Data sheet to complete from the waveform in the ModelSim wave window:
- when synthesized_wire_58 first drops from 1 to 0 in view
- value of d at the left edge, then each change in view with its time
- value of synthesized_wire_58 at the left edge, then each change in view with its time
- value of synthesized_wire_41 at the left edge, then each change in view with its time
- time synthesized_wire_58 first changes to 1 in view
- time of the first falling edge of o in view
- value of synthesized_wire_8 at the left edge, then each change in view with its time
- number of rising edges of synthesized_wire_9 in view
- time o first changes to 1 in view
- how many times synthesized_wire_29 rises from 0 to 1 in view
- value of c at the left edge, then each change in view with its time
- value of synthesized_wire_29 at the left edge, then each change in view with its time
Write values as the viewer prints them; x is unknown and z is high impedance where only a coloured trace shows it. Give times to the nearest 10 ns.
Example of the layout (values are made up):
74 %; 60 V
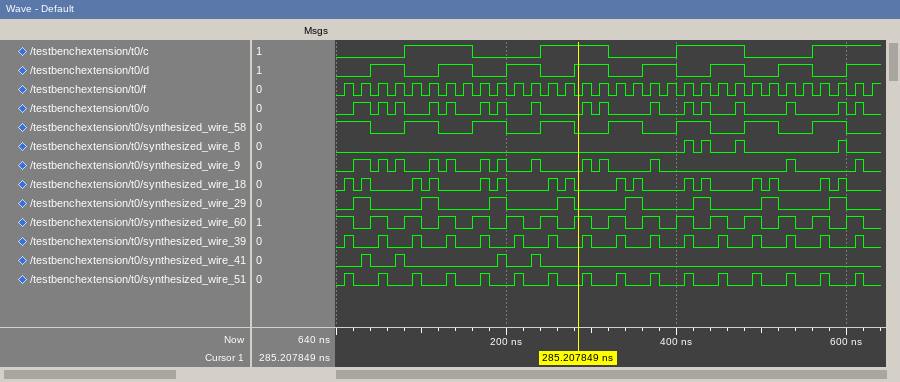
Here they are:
40 ns; 0, 1 at 40 ns, 0 at 80 ns, 1 at 120 ns, 0 at 160 ns, 1 at 200 ns, 0 at 240 ns, 1 at 280 ns, 0 at 320 ns, 1 at 360 ns, 0 at 400 ns, 1 at 440 ns, 0 at 480 ns, 1 at 520 ns, 0 at 560 ns, 1 at 600 ns; 1, 0 at 40 ns, 1 at 80 ns, 0 at 120 ns, 1 at 160 ns, 0 at 200 ns, 1 at 240 ns, 0 at 280 ns, 1 at 320 ns, 0 at 360 ns, 1 at 400 ns, 0 at 440 ns, 1 at 480 ns, 0 at 520 ns, 1 at 560 ns, 0 at 600 ns; 0, 1 at 30 ns, 0 at 40 ns, 1 at 70 ns, 0 at 80 ns, 1 at 190 ns, 0 at 200 ns, 1 at 230 ns, 0 at 240 ns; 80 ns; 40 ns; 0, 1 at 410 ns, 0 at 420 ns, 1 at 430 ns, 0 at 440 ns, 1 at 470 ns, 0 at 480 ns, 1 at 590 ns, 0 at 600 ns; 13; 20 ns; 8; 0, 1 at 80 ns, 0 at 160 ns, 1 at 240 ns, 0 at 320 ns, 1 at 400 ns, 0 at 480 ns, 1 at 560 ns; 0, 1 at 20 ns, 0 at 40 ns, 1 at 100 ns, 0 at 120 ns, 1 at 180 ns, 0 at 200 ns, 1 at 260 ns, 0 at 280 ns, 1 at 340 ns, 0 at 360 ns, 1 at 420 ns, 0 at 440 ns, 1 at 500 ns, 0 at 520 ns, 1 at 580 ns, 0 at 600 ns
